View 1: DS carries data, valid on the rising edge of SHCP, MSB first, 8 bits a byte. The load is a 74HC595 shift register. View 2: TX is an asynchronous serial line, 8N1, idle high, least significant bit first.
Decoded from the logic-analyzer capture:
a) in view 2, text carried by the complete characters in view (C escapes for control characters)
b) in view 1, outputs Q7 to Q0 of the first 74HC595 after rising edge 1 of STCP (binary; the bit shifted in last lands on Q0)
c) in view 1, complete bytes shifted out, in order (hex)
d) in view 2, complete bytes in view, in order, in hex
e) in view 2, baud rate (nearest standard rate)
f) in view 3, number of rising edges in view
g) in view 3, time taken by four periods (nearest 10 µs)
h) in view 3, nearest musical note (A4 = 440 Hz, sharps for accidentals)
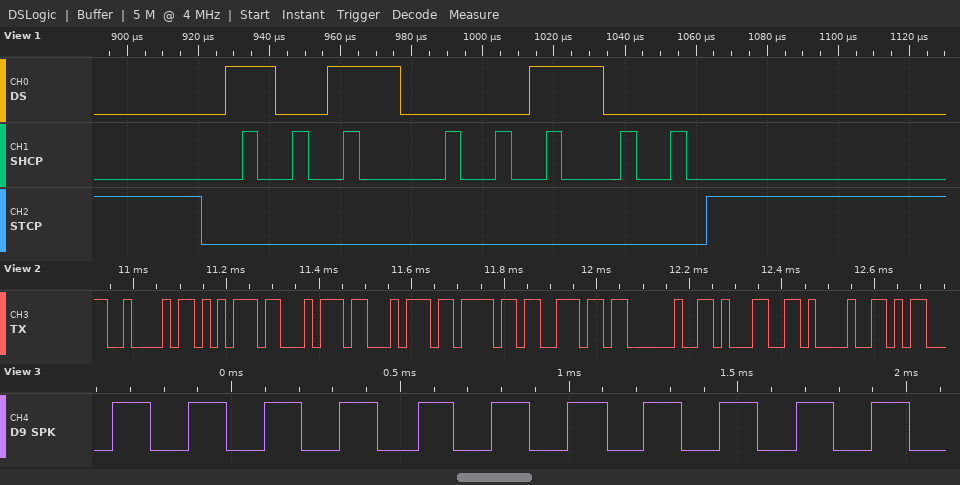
"Button 1!"
10100100
0xA4
42 75 74 74 6F 6E 20 31 21
57600 baud
11
900 µs
C#8
